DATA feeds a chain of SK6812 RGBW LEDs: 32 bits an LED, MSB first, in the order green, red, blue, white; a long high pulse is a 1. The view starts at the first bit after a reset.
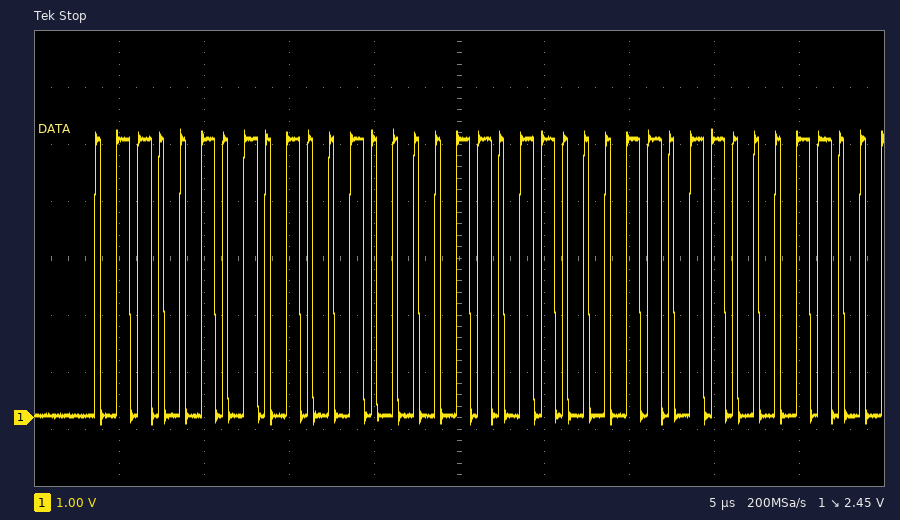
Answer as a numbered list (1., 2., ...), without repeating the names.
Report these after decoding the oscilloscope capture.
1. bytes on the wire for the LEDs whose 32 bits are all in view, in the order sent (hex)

1. 65 48 6C 6C
